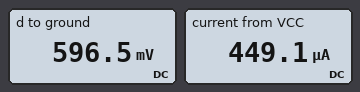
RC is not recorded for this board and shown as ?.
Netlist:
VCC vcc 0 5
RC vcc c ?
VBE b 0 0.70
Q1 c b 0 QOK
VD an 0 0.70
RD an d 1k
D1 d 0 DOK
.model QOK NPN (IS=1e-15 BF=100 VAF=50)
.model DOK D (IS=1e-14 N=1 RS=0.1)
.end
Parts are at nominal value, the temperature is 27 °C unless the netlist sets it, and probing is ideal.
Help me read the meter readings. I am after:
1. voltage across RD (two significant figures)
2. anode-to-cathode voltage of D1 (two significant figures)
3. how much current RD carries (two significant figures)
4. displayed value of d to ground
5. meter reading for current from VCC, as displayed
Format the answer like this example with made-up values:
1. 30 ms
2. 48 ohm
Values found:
1. 100 mV
2. 600 mV
3. 100 µA
4. 596.5 mV
5. 449.1 µA
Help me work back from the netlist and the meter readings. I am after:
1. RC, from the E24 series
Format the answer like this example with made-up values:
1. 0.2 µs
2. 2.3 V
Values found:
1. 11 kΩ
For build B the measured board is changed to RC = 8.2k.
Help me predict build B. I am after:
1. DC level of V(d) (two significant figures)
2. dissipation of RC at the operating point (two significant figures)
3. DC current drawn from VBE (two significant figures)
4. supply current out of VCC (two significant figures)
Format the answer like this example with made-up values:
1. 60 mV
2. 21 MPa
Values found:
1. 600 mV
2. 2.6 mW
3. 5.7 µA
4. 560 µA
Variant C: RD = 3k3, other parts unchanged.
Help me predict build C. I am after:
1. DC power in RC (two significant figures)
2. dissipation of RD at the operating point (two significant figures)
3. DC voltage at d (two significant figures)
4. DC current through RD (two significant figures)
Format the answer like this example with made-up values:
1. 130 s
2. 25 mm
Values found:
1. 2.2 mW
2. 5.0 µW
3. 570 mV
4. 39 µA
